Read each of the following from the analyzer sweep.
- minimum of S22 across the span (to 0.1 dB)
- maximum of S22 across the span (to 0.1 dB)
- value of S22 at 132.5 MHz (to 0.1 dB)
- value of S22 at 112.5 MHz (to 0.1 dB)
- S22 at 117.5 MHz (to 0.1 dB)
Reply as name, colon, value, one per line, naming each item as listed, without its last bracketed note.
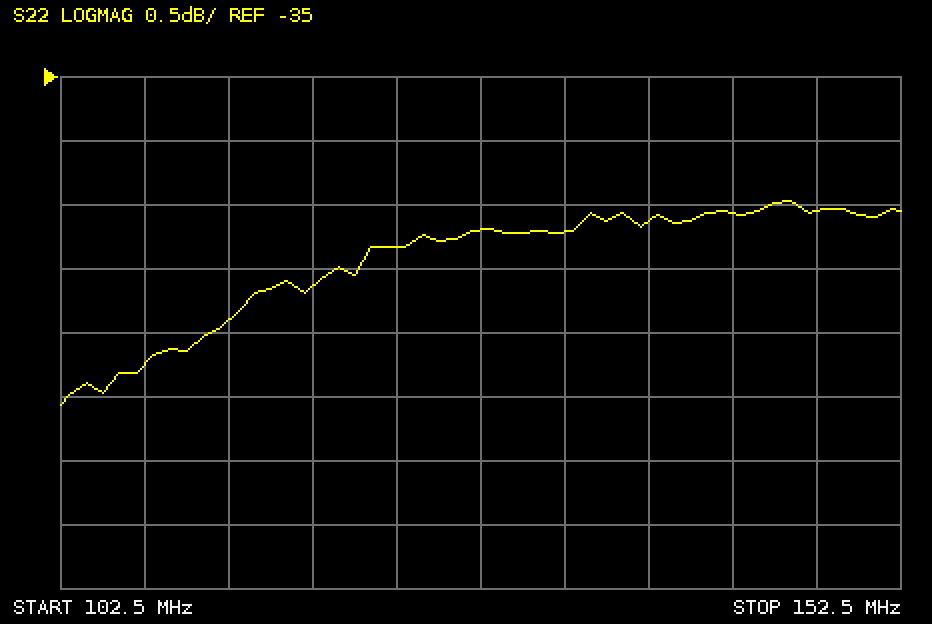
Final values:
minimum of S22 across the span: -37.6 dB
maximum of S22 across the span: -36.0 dB
value of S22 at 132.5 MHz: -36.2 dB
value of S22 at 112.5 MHz: -36.9 dB
S22 at 117.5 MHz: -36.6 dB
